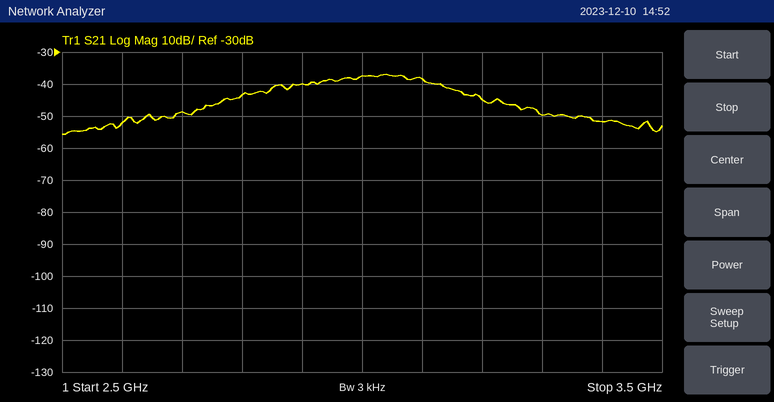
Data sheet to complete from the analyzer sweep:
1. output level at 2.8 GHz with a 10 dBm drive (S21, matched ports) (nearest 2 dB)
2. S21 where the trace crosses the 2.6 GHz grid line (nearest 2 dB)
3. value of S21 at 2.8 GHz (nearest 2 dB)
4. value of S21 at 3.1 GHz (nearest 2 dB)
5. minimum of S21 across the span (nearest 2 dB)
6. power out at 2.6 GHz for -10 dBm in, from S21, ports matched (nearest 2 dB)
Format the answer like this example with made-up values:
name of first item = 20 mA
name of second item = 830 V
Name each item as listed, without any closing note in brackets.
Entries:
output level at 2.8 GHz with a 10 dBm drive (S21, matched ports) = -34 dBm
S21 where the trace crosses the 2.6 GHz grid line = -52 dB
value of S21 at 2.8 GHz = -44 dB
value of S21 at 3.1 GHz = -38 dB
minimum of S21 across the span = -56 dB
power out at 2.6 GHz for -10 dBm in, from S21, ports matched = -62 dBm
